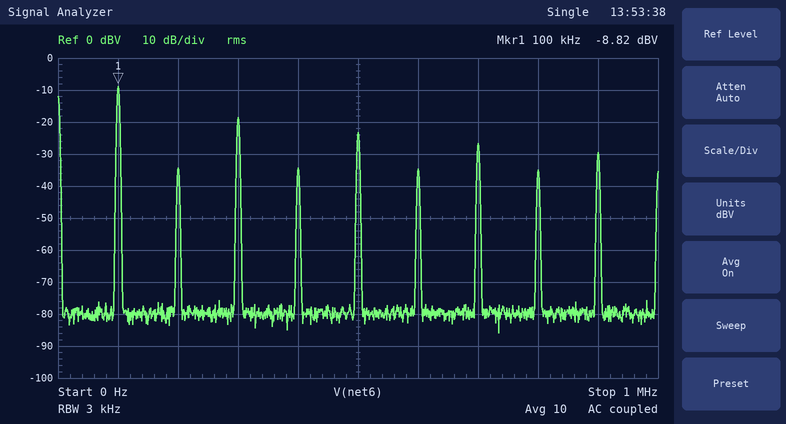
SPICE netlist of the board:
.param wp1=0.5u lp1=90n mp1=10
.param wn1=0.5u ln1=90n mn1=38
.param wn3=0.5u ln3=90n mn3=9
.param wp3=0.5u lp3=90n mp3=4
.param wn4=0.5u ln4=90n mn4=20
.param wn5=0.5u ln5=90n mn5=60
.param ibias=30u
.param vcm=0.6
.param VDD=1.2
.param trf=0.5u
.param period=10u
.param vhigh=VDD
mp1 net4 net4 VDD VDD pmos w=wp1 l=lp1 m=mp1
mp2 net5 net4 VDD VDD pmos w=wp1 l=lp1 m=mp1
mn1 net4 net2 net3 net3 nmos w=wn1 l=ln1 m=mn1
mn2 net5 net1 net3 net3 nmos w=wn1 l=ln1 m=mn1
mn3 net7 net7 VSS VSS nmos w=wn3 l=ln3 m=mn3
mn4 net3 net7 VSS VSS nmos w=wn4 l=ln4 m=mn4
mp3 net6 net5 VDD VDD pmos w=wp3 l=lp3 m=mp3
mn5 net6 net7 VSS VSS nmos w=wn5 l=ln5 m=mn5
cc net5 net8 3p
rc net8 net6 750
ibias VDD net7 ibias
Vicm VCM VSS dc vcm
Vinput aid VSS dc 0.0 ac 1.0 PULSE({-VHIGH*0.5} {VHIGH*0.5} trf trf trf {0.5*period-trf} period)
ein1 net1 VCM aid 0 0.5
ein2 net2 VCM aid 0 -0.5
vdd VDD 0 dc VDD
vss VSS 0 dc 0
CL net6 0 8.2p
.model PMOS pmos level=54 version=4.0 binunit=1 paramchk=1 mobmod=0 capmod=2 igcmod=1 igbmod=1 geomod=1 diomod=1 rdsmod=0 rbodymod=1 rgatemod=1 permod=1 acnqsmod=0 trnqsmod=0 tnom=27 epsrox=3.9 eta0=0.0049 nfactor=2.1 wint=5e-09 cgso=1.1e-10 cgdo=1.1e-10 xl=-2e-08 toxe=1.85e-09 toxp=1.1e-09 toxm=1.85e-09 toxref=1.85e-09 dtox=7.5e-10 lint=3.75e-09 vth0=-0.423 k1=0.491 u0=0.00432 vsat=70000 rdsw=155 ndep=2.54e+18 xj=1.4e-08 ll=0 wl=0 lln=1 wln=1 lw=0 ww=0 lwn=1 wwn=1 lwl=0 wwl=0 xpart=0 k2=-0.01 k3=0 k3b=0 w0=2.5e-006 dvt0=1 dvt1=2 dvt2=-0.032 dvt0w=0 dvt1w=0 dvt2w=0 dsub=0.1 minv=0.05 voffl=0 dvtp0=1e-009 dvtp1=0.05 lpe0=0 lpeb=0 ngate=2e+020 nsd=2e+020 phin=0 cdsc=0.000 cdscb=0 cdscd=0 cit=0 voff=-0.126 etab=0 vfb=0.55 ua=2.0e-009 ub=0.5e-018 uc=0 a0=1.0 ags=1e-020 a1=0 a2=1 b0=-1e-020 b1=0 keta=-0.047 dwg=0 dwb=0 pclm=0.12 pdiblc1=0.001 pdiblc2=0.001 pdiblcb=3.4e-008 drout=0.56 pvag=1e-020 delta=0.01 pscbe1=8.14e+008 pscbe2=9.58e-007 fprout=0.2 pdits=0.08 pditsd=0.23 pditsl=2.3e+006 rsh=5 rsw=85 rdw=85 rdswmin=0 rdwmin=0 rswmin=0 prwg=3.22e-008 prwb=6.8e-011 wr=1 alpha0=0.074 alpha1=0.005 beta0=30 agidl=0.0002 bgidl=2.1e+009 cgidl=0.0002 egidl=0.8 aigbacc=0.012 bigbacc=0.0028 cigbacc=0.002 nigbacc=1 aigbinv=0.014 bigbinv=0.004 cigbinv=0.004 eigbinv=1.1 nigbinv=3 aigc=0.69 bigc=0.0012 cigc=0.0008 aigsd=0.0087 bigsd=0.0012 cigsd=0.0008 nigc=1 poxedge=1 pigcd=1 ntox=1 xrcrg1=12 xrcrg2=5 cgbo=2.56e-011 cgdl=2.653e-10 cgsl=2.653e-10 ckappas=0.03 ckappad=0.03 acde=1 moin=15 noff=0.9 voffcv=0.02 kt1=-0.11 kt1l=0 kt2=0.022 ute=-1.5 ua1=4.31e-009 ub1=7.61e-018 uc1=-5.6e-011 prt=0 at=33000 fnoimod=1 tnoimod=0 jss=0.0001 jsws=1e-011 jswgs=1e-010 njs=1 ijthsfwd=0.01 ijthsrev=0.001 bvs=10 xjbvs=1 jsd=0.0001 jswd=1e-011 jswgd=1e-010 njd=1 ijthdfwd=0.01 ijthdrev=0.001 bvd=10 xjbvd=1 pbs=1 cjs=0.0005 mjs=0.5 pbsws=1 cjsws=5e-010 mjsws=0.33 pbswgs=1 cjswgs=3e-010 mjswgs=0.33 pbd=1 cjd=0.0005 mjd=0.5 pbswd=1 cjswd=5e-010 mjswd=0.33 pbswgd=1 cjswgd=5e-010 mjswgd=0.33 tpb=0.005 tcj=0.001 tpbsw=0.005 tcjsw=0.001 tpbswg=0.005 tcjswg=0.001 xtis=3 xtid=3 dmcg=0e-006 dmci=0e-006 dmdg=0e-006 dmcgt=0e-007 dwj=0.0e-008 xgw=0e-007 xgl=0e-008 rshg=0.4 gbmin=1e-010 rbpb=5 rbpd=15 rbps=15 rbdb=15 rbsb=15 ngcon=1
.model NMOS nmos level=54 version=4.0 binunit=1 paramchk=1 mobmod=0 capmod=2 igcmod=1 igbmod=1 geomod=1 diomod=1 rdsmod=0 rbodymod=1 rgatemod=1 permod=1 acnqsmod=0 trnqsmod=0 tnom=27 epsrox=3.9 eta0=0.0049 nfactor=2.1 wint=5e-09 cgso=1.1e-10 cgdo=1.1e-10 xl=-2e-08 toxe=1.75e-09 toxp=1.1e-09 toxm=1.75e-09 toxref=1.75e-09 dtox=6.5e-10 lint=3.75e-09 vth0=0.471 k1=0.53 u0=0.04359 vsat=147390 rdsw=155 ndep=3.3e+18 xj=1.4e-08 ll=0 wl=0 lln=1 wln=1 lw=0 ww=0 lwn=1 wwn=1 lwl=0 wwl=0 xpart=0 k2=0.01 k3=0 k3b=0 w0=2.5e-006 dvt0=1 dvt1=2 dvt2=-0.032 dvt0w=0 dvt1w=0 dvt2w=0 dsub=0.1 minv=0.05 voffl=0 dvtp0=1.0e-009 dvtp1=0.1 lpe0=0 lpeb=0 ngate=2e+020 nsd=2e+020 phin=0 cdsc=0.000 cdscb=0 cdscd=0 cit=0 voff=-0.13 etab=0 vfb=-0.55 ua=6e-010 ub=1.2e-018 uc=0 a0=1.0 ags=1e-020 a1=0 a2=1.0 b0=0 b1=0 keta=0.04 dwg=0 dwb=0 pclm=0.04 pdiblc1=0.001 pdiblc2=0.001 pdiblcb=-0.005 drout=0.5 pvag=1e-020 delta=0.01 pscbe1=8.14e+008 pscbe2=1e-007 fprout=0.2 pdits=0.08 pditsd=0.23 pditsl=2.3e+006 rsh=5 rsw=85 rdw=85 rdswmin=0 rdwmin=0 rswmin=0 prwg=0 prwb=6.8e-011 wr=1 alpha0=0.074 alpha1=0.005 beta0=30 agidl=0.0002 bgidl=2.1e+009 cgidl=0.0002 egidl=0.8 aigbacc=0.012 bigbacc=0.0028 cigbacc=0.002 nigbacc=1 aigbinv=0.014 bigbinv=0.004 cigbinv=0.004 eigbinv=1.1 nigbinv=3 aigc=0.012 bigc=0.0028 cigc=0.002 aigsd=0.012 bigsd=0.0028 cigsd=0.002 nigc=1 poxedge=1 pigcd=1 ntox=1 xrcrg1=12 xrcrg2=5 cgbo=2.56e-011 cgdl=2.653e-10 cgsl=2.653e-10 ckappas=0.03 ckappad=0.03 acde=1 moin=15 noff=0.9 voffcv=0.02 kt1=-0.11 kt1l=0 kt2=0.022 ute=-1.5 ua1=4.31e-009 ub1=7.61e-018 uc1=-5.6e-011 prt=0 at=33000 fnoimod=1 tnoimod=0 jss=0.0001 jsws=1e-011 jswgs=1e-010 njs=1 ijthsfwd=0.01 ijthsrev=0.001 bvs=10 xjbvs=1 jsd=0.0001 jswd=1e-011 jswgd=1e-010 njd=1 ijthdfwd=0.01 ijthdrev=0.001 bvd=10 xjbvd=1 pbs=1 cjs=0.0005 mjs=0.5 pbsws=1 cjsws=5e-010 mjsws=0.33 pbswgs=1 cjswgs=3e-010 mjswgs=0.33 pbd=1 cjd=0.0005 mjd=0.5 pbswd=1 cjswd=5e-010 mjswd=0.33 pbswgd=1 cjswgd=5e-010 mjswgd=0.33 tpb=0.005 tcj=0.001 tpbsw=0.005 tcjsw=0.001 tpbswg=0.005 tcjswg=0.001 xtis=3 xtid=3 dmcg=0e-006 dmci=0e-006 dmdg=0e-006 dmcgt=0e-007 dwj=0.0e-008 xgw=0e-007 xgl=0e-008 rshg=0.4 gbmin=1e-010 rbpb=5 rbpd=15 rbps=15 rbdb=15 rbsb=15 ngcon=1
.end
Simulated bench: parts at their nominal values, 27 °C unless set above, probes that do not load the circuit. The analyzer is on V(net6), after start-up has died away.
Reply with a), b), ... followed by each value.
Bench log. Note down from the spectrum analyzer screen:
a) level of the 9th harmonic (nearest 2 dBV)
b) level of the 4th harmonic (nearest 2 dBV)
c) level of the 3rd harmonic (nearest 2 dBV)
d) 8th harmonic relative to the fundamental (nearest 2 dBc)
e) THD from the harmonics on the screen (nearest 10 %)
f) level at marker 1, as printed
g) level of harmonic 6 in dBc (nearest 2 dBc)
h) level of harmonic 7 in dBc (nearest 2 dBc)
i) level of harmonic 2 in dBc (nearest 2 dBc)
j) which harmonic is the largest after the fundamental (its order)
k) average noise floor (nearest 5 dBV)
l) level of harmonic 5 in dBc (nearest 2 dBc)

a) -30 dBV
b) -34 dBV
c) -18 dBV
d) -26 dBc
e) 40 %
f) -8.82 dBV
g) -26 dBc
h) -18 dBc
i) -26 dBc
j) 3
k) -80 dBV
l) -14 dBc
